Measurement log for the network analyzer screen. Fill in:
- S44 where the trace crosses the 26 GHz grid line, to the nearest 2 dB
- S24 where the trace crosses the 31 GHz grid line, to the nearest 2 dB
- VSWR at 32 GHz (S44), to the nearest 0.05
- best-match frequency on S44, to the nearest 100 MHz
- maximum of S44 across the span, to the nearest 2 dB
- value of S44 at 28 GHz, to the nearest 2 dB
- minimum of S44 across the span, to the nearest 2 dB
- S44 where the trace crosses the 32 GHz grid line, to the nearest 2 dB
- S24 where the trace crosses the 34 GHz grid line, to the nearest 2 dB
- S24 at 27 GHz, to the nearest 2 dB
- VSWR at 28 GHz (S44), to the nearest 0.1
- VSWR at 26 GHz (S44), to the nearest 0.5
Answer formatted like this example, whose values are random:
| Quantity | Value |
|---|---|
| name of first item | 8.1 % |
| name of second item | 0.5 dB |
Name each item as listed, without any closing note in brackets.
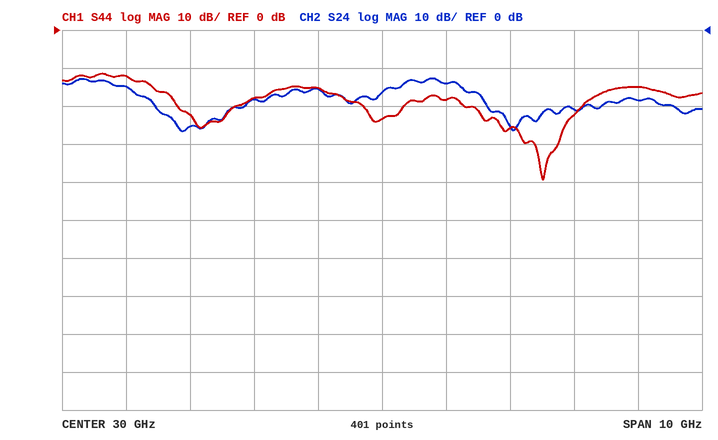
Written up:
| Quantity | Value |
|---|---|
| S44 where the trace crosses the 26 GHz grid line, to the nearest 2 dB | -12 dB |
| S24 where the trace crosses the 31 GHz grid line, to the nearest 2 dB | -14 dB |
| VSWR at 32 GHz (S44), to the nearest 0.05 | 1.10 |
| best-match frequency on S44, to the nearest 100 MHz | 32.5 GHz |
| maximum of S44 across the span, to the nearest 2 dB | -12 dB |
| value of S44 at 28 GHz, to the nearest 2 dB | -18 dB |
| minimum of S44 across the span, to the nearest 2 dB | -40 dB |
| S44 where the trace crosses the 32 GHz grid line, to the nearest 2 dB | -26 dB |
| S24 where the trace crosses the 34 GHz grid line, to the nearest 2 dB | -18 dB |
| S24 at 27 GHz, to the nearest 2 dB | -26 dB |
| VSWR at 28 GHz (S44), to the nearest 0.1 | 1.3 |
| VSWR at 26 GHz (S44), to the nearest 0.5 | 1.5 |
